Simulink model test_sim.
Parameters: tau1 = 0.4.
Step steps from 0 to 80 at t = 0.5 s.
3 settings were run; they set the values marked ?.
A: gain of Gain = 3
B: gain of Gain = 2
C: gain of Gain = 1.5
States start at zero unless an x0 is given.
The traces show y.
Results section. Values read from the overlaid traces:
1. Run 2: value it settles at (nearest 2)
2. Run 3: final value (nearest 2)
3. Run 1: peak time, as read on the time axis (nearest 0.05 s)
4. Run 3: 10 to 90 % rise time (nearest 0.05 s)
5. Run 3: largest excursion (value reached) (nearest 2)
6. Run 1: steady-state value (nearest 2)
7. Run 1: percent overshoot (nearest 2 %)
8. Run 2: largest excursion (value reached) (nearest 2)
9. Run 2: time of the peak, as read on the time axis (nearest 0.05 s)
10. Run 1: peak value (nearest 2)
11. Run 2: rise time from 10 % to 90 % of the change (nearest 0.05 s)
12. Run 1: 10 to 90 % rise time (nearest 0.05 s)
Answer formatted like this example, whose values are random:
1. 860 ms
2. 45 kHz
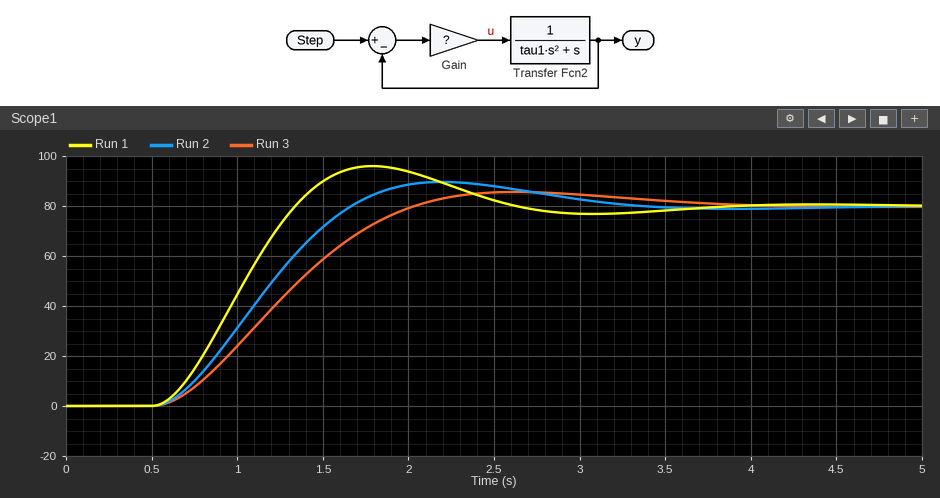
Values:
1. 80
2. 80
3. 1.80 s
4. 1.00 s
5. 86
6. 80
7. 20 %
8. 90
9. 2.20 s
10. 96
11. 0.80 s
12. 0.55 s
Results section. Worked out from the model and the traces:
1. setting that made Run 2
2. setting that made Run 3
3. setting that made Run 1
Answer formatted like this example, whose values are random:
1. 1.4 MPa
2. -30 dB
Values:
1. B
2. C
3. A
